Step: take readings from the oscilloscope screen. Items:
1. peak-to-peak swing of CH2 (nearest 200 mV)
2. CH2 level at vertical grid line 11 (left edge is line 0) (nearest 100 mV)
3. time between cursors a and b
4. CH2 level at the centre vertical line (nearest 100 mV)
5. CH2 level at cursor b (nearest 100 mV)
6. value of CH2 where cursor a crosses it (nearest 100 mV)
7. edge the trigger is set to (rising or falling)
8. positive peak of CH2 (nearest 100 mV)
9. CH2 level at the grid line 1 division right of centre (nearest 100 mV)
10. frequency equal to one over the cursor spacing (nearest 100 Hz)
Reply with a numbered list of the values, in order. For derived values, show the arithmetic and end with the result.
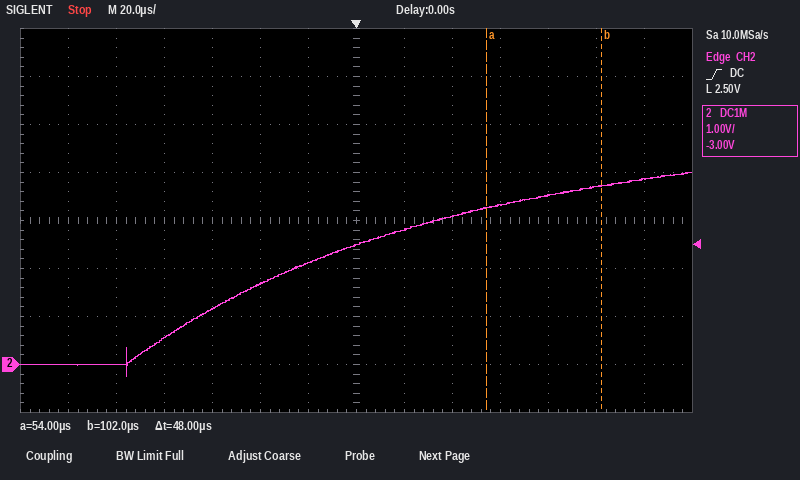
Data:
1. 4.2 V
2. 3.5 V
3. 48 µs
4. 2.5 V
5. 3.7 V
6. 3.3 V
7. rising
8. 4.0 V
9. 2.8 V
10. 1 / 48 µs ≈ 20.8 kHz
